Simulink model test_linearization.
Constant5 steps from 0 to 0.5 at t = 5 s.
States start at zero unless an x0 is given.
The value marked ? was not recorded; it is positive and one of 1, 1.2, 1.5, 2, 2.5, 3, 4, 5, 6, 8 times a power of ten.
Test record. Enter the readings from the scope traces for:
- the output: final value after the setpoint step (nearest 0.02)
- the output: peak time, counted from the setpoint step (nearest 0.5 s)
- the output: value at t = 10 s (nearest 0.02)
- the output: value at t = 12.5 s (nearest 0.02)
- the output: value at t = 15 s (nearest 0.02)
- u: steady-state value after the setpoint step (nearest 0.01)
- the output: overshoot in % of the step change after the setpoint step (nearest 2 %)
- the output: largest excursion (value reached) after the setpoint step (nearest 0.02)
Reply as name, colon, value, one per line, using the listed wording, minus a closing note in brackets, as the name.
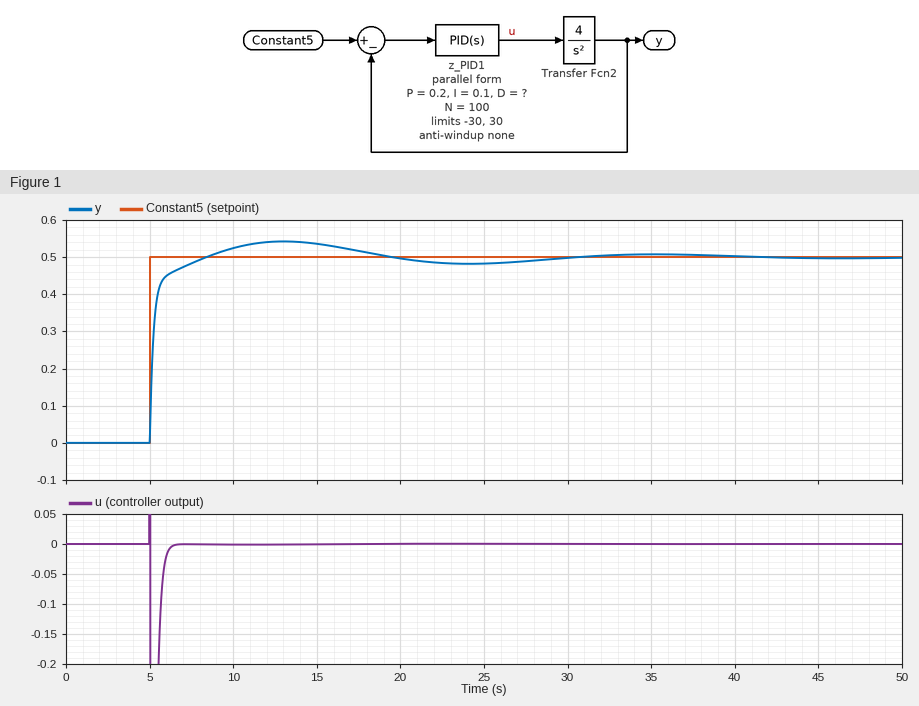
the output: final value after the setpoint step: 0.50
the output: peak time, counted from the setpoint step: 8.0 s
the output: value at t = 10 s: 0.52
the output: value at t = 12.5 s: 0.54
the output: value at t = 15 s: 0.54
u: steady-state value after the setpoint step: 0.00
the output: overshoot in % of the step change after the setpoint step: 8 %
the output: largest excursion (value reached) after the setpoint step: 0.54
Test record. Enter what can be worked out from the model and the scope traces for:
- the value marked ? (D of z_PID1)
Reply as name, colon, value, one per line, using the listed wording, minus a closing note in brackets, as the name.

the value marked ?: 1.2
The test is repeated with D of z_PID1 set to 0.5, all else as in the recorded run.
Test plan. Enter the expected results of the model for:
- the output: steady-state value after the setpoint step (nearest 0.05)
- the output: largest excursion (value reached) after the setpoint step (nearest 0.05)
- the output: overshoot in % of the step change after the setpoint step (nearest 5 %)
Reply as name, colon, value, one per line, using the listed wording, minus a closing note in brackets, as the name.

the output: steady-state value after the setpoint step: 0.50
the output: largest excursion (value reached) after the setpoint step: 0.60
the output: overshoot in % of the step change after the setpoint step: 20 %
